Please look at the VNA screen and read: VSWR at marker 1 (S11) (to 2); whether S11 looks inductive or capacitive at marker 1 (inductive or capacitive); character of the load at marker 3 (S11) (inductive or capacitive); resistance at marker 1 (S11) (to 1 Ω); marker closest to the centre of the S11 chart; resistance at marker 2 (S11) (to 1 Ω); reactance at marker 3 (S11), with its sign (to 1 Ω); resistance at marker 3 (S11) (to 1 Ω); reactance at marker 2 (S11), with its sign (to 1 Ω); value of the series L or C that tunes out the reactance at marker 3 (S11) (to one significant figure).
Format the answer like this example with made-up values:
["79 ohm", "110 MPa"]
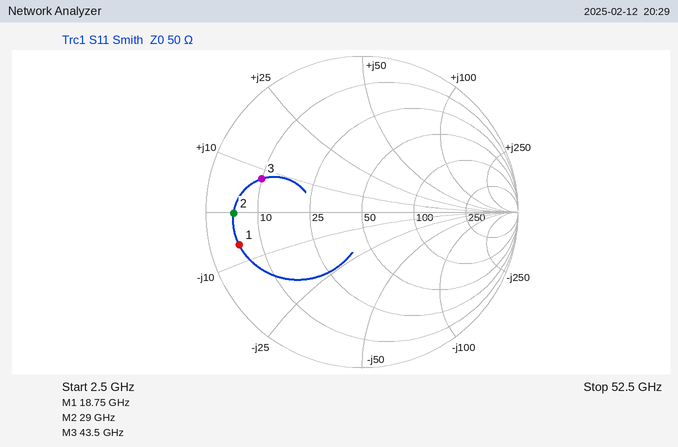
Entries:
["10", "capacitive", "inductive", "5 Ω", "marker 3", "5 Ω", "+8 Ω", "10 Ω", "0 Ω", "500 fF"]
